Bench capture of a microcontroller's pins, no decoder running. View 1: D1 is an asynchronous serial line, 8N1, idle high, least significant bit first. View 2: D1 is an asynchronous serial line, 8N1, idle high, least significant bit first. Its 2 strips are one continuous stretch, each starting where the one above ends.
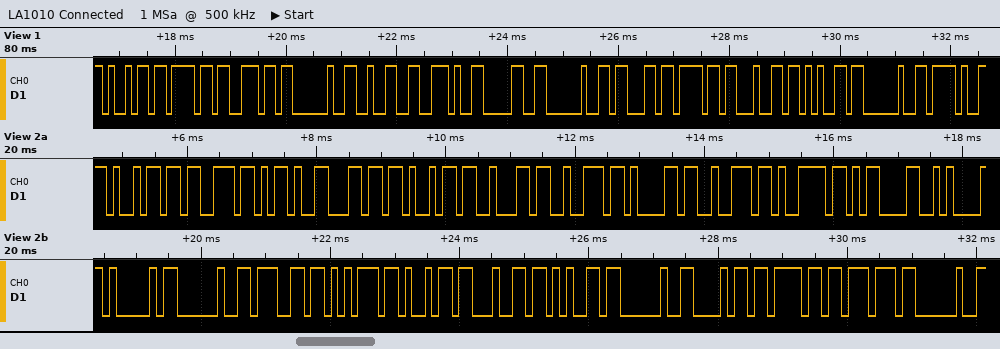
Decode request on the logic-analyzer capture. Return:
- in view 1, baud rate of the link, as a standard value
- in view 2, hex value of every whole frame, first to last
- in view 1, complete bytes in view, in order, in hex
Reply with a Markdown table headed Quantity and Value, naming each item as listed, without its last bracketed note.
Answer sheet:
| Quantity | Value |
|---|---|
| in view 1, baud rate of the link, as a standard value | 9600 baud |
| in view 2, hex value of every whole frame, first to last | 69 73 2D 6C 69 62 72 61 72 79 0D 0A 41 20 67 75 69 64 65 20 68 6F 77 20 |
| in view 1, complete bytes in view, in order, in hex | 69 6F 6E 20 32 2E 30 20 63 6F 64 65 20 2F |
